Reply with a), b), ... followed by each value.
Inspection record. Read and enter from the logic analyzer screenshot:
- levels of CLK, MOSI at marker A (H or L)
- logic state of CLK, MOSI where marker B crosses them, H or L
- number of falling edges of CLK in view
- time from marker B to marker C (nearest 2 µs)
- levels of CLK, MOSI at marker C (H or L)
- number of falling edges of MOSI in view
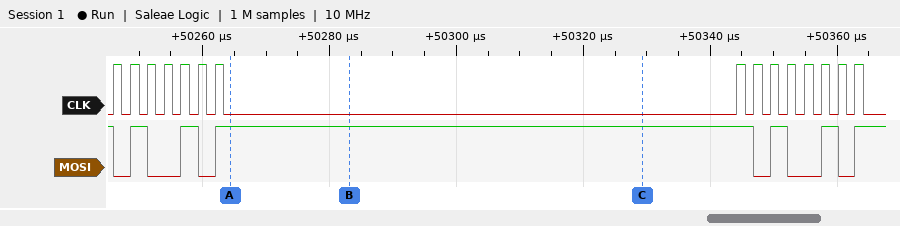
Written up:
a) CLK=L, MOSI=H
b) CLK=L, MOSI=H
c) 15
d) 46 µs
e) CLK=L, MOSI=H
f) 6
